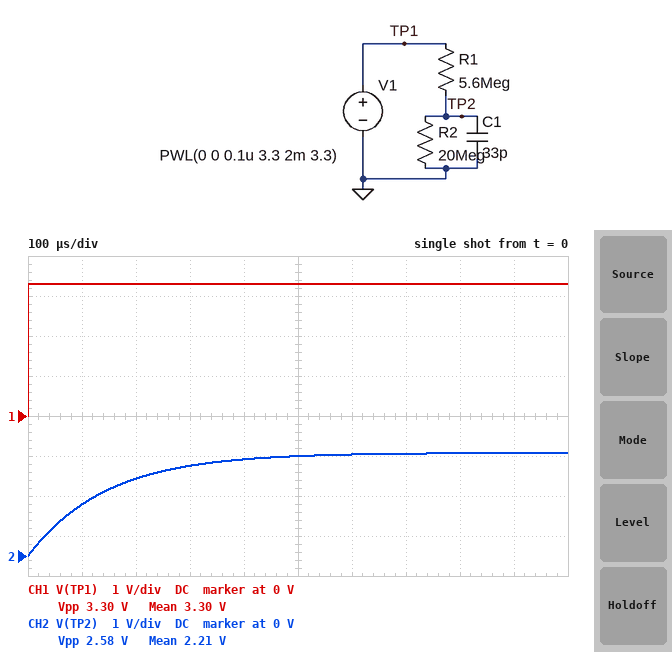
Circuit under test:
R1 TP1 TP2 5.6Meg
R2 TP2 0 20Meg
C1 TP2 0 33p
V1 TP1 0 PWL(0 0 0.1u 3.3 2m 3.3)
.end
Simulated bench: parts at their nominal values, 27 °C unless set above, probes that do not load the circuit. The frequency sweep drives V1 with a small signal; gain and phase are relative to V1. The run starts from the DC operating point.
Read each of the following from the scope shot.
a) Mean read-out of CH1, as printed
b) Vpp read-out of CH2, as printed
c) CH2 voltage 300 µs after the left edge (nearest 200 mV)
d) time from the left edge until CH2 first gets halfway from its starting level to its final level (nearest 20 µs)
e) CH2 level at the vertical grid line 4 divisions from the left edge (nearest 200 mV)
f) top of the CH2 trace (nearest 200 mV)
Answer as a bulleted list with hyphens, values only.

- 3.30 V
- 2.58 V
- 2.2 V
- 100 µs
- 2.4 V
- 2.6 V
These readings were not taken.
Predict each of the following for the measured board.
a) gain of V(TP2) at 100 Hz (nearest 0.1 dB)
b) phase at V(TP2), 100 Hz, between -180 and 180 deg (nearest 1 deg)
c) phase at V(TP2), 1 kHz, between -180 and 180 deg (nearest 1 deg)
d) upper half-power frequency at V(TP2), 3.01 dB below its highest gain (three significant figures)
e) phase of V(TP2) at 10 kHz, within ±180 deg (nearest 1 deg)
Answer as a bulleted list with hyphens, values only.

- -2.2 dB
- -5 deg
- -42 deg
- 1.10 kHz
- -84 deg
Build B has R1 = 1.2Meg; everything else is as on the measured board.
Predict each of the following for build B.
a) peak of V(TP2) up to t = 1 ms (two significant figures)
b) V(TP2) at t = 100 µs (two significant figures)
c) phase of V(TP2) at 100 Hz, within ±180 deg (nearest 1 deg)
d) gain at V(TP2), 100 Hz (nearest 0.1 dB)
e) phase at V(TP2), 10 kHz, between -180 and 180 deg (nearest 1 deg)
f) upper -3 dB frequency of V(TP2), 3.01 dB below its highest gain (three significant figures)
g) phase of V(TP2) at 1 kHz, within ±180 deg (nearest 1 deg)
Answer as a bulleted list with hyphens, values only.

- 3.1 V
- 2.9 V
- -1 deg
- -0.5 dB
- -67 deg
- 4.26 kHz
- -13 deg
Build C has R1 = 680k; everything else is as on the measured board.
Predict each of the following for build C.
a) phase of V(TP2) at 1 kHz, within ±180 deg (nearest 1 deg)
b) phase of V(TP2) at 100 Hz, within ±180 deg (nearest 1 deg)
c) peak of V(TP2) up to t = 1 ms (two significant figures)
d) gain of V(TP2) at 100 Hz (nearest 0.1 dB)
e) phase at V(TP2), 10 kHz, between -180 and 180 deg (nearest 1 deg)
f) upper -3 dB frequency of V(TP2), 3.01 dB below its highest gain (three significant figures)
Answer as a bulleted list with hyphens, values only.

- -8 deg
- -1 deg
- 3.2 V
- -0.3 dB
- -54 deg
- 7.33 kHz
